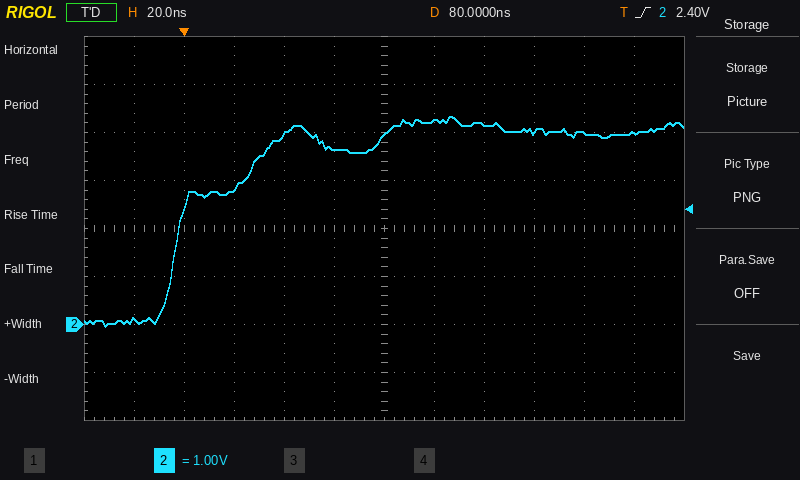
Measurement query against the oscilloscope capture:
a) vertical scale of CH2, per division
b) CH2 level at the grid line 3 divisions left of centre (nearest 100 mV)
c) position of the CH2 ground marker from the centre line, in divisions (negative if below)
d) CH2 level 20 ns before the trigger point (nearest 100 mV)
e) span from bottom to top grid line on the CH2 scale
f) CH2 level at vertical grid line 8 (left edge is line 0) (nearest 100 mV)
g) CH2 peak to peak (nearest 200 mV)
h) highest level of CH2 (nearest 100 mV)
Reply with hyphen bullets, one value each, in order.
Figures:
- 1 V
- 2.8 V
- -2.0 div
- 100 mV
- 8 V
- 4.2 V
- 4.4 V
- 4.3 V
